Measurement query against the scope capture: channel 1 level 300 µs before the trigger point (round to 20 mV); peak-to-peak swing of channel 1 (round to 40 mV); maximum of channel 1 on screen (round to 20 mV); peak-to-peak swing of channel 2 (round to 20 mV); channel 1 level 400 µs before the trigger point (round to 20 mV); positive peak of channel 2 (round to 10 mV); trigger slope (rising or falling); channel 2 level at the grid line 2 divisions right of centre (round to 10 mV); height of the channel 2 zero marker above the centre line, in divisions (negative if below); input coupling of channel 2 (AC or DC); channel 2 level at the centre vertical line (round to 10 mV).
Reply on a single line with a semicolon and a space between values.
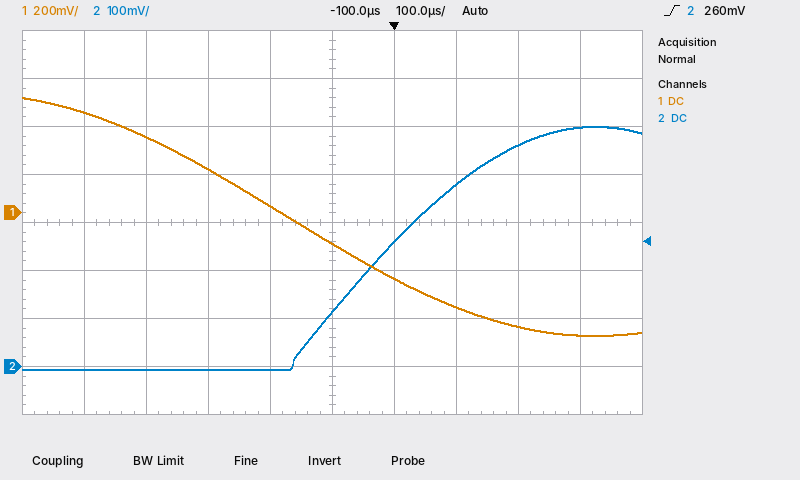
180 mV; 1.00 V; 480 mV; 500 mV; 320 mV; 500 mV; rising; 380 mV; -3.0 div; DC; 110 mV
